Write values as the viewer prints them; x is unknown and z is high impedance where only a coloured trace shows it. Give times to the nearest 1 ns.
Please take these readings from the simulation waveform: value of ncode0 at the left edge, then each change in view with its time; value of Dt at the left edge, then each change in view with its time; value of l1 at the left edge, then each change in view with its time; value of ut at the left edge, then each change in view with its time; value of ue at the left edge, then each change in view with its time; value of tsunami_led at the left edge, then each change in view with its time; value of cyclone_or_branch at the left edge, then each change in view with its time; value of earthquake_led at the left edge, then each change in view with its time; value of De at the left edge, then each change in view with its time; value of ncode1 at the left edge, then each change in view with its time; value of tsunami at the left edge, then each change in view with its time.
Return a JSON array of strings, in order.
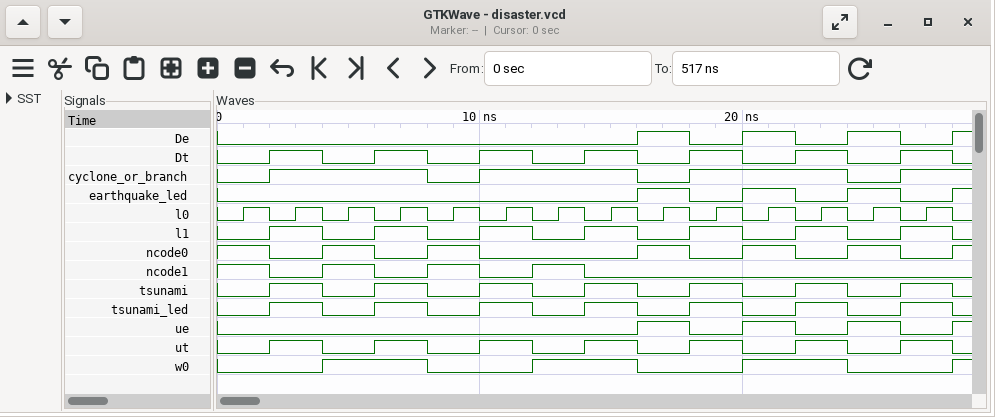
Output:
["1, 0 at 2 ns, 1 at 4 ns, 0 at 6 ns, 1 at 8 ns, 0 at 10 ns, 1 at 16 ns, 0 at 18 ns, 1 at 20 ns, 0 at 22 ns, 1 at 24 ns, 0 at 26 ns, 1 at 28 ns", "0, 1 at 2 ns, 0 at 4 ns, 1 at 6 ns, 0 at 8 ns, 1 at 10 ns, 0 at 12 ns, 1 at 14 ns, 0 at 16 ns, 1 at 18 ns, 0 at 20 ns, 1 at 22 ns, 0 at 24 ns, 1 at 26 ns, 0 at 28 ns", "0, 1 at 2 ns, 0 at 4 ns, 1 at 6 ns, 0 at 8 ns, 1 at 10 ns, 0 at 12 ns, 1 at 14 ns, 0 at 16 ns, 1 at 18 ns, 0 at 20 ns, 1 at 22 ns, 0 at 24 ns, 1 at 26 ns, 0 at 28 ns", "0, 1 at 2 ns, 0 at 4 ns, 1 at 6 ns, 0 at 8 ns, 1 at 10 ns, 0 at 12 ns, 1 at 14 ns, 0 at 16 ns, 1 at 18 ns, 0 at 20 ns, 1 at 22 ns, 0 at 24 ns, 1 at 26 ns, 0 at 28 ns", "0, 1 at 16 ns, 0 at 18 ns, 1 at 20 ns, 0 at 22 ns, 1 at 24 ns, 0 at 26 ns, 1 at 28 ns", "0, 1 at 2 ns, 0 at 4 ns, 1 at 6 ns, 0 at 8 ns, 1 at 10 ns, 0 at 12 ns, 1 at 14 ns, 0 at 16 ns, 1 at 18 ns, 0 at 20 ns, 1 at 22 ns, 0 at 24 ns, 1 at 26 ns, 0 at 28 ns", "0, 1 at 2 ns, 0 at 8 ns, 1 at 10 ns, 0 at 16 ns, 1 at 18 ns, 0 at 24 ns, 1 at 26 ns", "0, 1 at 16 ns, 0 at 18 ns, 1 at 20 ns, 0 at 22 ns, 1 at 24 ns, 0 at 26 ns, 1 at 28 ns", "0, 1 at 16 ns, 0 at 18 ns, 1 at 20 ns, 0 at 22 ns, 1 at 24 ns, 0 at 26 ns, 1 at 28 ns", "1, 0 at 2 ns, 1 at 4 ns, 0 at 6 ns, 1 at 8 ns, 0 at 10 ns, 1 at 12 ns, 0 at 14 ns", "0, 1 at 2 ns, 0 at 4 ns, 1 at 6 ns, 0 at 8 ns, 1 at 10 ns, 0 at 12 ns, 1 at 14 ns, 0 at 16 ns, 1 at 18 ns, 0 at 20 ns, 1 at 22 ns, 0 at 24 ns, 1 at 26 ns, 0 at 28 ns"]
